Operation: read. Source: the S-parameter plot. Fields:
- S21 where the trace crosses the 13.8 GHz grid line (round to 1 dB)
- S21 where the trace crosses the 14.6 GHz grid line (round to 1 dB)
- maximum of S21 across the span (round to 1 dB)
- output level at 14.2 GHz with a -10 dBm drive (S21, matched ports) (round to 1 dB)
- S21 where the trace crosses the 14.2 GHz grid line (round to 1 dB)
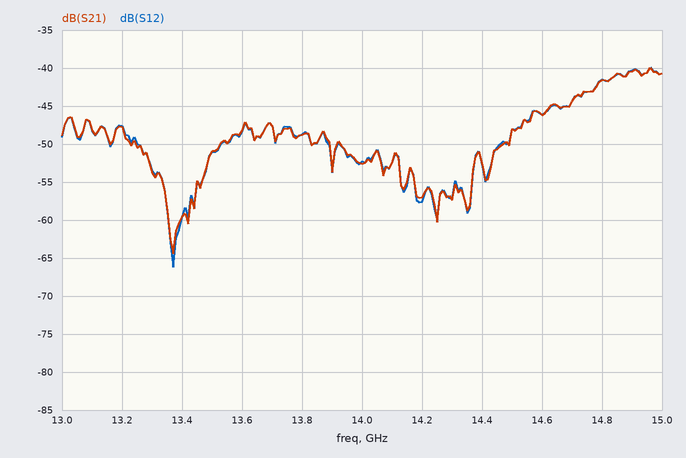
-49 dB
-46 dB
-40 dB
-67 dBm
-57 dB
